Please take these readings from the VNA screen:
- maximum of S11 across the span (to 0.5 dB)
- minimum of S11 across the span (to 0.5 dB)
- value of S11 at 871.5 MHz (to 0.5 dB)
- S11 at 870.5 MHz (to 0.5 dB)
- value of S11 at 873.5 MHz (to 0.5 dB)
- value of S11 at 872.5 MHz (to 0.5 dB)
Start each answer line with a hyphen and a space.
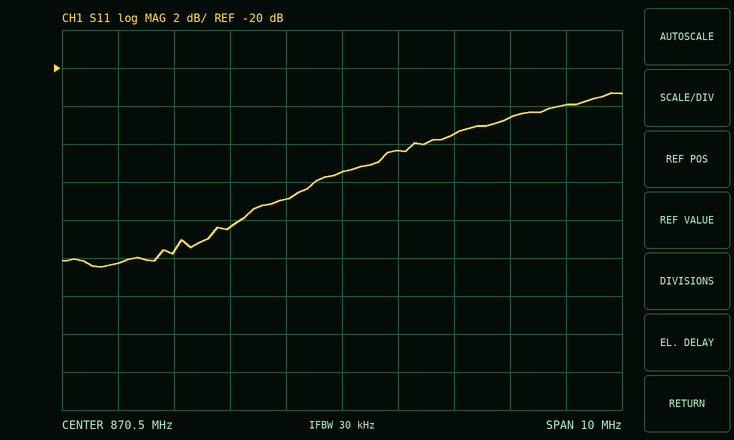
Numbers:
- -21.5 dB
- -30.5 dB
- -24.5 dB
- -25.5 dB
- -22.5 dB
- -23.5 dB
